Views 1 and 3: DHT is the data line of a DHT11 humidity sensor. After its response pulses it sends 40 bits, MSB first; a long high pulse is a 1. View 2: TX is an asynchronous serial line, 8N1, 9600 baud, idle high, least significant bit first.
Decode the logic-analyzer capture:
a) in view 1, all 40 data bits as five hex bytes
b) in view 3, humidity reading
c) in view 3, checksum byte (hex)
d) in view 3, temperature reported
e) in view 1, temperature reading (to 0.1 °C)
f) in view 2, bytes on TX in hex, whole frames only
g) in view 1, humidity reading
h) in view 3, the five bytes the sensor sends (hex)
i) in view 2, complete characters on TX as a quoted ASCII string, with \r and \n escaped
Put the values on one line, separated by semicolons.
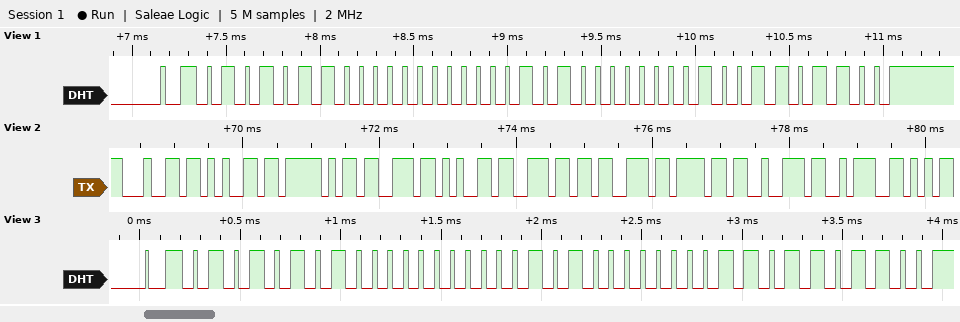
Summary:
56 00 14 02 6C; 85 %; 0x6C; 20.3 °C; 20.2 °C; 64 65 5F 73 65 6E 73 6F 72 3A; 86 %; 55 00 14 03 6C; "de_sensor:"
